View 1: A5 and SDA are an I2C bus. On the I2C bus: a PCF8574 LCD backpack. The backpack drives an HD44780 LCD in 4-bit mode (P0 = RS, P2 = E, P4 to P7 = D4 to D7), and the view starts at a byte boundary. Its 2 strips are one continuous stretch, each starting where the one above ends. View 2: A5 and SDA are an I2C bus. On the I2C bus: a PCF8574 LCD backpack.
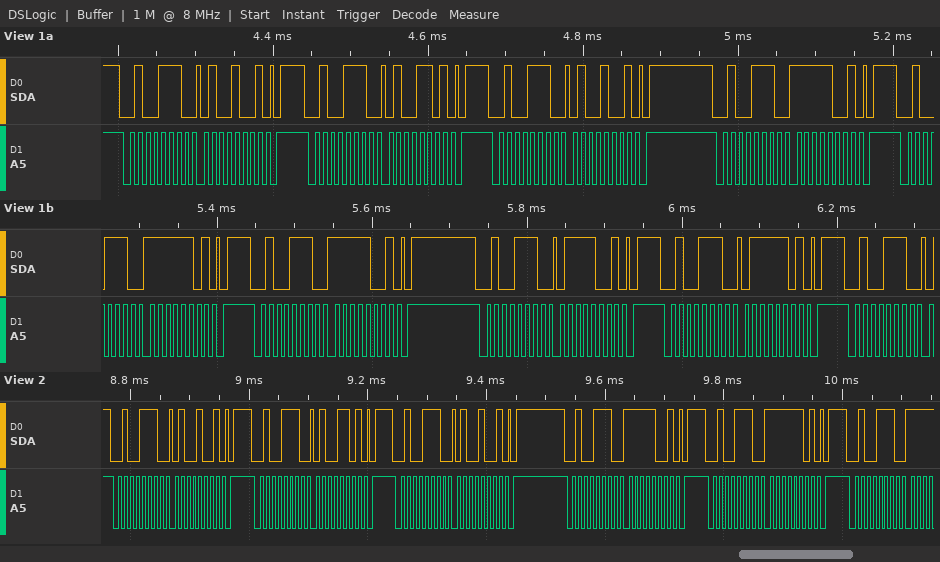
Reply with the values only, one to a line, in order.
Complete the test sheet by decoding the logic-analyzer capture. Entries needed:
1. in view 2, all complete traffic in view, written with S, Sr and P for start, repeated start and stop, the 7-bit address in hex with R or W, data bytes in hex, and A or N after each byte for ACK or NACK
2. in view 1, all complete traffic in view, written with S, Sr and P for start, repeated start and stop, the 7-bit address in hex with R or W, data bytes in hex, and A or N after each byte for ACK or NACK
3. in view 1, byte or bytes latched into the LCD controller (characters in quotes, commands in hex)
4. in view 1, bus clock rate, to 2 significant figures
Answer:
S 27W A 49 A P S 27W A 4D A P S 27W A 49 A P S 27W A F9 A P S 27W A FD A P S 27W A
S 27W A 49 A P S 27W A 4D A P S 27W A 49 A P S 27W A F9 A P S 27W A FD A P S 27W A F9 A P S 27W A 79 A P S 27W A 7D A P S 27W A
'O'
100 kHz
